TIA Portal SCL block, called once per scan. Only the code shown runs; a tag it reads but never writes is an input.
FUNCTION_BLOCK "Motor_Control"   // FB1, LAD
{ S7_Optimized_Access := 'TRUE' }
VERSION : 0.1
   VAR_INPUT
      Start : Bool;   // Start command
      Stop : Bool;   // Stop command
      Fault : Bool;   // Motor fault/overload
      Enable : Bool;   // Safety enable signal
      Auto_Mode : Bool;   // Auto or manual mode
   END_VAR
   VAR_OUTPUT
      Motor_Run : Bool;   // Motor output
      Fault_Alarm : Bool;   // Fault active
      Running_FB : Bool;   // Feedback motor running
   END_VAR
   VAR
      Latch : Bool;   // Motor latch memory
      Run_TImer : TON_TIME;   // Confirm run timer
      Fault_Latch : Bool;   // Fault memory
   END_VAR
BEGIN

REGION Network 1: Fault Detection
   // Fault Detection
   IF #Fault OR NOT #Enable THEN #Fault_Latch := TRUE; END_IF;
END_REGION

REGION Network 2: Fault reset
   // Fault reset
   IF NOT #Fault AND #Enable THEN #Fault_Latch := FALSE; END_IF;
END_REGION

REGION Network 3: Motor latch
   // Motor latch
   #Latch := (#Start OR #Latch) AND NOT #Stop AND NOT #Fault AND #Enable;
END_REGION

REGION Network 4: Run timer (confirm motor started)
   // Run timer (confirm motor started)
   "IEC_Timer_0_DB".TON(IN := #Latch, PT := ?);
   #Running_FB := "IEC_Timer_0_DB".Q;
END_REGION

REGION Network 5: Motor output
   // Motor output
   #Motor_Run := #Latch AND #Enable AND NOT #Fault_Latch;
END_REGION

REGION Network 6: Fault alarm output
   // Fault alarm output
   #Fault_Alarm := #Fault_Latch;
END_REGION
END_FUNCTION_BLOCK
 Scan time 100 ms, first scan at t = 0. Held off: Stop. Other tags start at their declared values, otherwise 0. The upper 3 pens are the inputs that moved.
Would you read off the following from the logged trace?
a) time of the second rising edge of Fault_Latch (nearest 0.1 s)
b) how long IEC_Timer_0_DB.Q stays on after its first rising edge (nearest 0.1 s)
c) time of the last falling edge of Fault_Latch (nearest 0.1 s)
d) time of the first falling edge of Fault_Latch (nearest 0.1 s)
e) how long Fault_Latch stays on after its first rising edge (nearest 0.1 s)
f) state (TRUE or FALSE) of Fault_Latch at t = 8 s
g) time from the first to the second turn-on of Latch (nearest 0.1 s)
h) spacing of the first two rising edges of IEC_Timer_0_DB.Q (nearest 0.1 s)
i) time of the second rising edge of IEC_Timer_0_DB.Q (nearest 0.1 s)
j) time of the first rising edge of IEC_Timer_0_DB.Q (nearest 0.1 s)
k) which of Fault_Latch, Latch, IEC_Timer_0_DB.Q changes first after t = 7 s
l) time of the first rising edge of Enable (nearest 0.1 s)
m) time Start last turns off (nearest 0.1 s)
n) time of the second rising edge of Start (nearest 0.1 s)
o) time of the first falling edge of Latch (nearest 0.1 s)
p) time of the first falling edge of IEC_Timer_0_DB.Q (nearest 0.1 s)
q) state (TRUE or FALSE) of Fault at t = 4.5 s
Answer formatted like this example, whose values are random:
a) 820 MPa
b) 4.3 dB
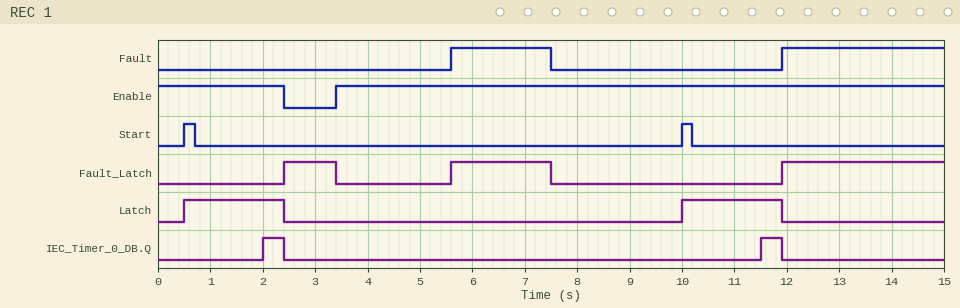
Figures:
a) 5.6 s
b) 0.4 s
c) 7.5 s
d) 3.4 s
e) 1.0 s
f) FALSE
g) 9.5 s
h) 9.5 s
i) 11.5 s
j) 2.0 s
k) Fault_Latch
l) 3.4 s
m) 10.2 s
n) 10.0 s
o) 2.4 s
p) 2.4 s
q) FALSE
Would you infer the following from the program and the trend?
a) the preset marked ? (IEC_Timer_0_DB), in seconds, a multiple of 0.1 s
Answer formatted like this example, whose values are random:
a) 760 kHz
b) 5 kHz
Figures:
a) 1.5 s
